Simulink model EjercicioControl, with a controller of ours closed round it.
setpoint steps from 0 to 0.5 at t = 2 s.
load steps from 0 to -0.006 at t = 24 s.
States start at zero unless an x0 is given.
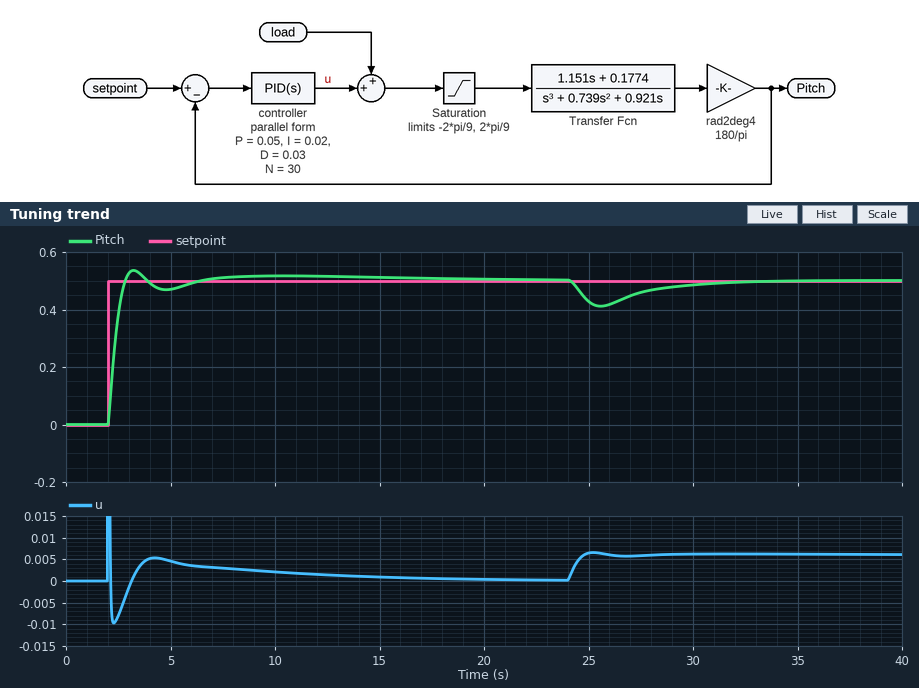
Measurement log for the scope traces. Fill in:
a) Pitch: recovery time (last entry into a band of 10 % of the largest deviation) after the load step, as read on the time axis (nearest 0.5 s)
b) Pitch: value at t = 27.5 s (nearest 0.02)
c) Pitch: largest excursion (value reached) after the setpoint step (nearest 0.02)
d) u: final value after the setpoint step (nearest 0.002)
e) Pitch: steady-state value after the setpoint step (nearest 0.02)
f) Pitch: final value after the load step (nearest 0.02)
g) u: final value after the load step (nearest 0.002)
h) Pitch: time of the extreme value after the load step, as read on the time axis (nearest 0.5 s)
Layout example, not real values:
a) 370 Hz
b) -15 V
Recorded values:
a) 31.0 s
b) 0.46
c) 0.54
d) 0.000
e) 0.50
f) 0.50
g) 0.006
h) 25.5 s
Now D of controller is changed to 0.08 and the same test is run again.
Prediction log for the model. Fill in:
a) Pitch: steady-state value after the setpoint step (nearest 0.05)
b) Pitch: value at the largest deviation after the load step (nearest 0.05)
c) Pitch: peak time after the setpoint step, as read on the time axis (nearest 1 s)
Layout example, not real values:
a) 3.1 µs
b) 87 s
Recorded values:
a) 0.50
b) 0.45
c) 10 s
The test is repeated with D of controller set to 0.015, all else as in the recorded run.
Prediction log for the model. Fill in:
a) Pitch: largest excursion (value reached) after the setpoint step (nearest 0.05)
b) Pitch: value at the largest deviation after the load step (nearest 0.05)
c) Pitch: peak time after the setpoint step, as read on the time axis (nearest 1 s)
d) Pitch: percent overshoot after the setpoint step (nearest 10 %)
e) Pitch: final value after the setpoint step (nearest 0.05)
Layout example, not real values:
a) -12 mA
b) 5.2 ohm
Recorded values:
a) 0.60
b) 0.40
c) 3 s
d) 20 %
e) 0.50
